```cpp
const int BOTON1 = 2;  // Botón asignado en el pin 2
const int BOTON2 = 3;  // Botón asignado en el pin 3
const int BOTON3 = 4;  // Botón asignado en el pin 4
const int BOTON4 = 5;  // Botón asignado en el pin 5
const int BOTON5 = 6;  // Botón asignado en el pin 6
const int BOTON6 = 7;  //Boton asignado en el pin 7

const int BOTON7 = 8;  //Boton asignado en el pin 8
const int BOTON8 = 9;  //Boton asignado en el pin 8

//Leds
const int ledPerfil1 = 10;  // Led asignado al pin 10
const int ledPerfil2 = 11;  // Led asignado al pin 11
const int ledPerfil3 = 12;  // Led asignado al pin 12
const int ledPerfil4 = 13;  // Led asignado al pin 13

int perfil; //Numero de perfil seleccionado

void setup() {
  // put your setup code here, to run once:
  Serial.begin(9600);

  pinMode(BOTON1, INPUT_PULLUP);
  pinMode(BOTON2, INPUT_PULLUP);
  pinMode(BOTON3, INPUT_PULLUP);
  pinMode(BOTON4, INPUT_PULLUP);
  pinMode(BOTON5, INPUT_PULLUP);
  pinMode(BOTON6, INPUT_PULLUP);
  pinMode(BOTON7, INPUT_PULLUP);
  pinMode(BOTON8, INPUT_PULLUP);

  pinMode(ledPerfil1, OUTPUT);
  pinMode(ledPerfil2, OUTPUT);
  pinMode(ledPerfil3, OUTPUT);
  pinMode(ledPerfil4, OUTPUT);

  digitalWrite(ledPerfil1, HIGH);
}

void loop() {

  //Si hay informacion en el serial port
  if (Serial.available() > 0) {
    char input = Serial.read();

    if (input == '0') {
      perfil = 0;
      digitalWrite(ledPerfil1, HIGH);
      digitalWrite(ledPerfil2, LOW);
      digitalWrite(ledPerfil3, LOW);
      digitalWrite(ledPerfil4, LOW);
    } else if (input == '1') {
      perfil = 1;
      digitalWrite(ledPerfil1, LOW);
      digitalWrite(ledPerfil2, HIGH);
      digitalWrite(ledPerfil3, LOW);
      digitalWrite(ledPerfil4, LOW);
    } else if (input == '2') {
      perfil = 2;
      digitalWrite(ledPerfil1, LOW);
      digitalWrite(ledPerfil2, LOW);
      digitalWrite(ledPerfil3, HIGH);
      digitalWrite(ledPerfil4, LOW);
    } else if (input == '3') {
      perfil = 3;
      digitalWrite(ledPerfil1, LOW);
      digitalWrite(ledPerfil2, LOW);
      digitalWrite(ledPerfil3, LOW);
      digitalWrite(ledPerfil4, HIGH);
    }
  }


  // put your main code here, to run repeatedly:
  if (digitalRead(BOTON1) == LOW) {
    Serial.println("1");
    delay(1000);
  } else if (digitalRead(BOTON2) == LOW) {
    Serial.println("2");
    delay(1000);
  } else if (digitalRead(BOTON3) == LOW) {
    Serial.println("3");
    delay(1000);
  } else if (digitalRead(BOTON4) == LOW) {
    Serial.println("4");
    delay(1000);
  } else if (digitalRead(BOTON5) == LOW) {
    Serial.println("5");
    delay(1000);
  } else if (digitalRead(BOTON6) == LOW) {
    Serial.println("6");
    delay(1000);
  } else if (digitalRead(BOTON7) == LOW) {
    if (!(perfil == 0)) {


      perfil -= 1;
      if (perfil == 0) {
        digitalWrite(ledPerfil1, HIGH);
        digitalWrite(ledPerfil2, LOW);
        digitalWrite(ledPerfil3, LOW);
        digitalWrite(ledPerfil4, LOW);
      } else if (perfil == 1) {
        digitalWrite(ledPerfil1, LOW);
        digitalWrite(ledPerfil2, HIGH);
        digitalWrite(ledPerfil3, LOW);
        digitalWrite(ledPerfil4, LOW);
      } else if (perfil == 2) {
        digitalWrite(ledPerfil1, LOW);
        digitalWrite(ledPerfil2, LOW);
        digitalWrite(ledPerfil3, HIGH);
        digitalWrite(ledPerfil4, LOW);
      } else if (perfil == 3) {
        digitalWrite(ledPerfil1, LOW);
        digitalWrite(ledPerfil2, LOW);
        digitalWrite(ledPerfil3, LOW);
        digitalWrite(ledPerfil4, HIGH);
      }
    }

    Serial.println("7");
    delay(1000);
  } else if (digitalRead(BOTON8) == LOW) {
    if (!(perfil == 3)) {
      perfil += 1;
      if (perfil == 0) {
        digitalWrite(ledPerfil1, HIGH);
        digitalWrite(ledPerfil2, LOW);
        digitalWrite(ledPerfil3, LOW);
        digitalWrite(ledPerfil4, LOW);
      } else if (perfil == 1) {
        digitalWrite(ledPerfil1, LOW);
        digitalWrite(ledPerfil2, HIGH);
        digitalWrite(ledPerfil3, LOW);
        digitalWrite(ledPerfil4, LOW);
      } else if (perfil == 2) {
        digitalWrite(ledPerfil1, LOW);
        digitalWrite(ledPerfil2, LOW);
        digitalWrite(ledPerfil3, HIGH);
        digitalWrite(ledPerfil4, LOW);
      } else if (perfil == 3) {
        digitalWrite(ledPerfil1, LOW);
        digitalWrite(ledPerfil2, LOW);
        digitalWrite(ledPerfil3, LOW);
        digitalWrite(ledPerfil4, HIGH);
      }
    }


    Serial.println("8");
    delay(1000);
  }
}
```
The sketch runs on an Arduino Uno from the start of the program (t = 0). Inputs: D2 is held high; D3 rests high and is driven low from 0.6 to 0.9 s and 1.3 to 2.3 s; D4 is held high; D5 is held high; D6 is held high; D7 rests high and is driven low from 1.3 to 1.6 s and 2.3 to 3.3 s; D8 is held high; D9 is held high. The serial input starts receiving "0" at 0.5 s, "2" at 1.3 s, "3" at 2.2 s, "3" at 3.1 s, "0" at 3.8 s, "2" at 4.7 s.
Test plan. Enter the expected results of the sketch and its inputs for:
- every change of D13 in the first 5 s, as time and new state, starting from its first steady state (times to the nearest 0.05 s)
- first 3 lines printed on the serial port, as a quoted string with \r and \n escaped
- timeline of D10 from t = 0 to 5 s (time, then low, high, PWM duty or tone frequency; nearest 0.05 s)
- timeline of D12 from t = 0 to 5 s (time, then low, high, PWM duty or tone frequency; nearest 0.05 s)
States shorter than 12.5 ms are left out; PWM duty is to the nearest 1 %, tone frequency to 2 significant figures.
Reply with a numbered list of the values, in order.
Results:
1. 0 s low; 2.6 s high; 3.8 s low
2. "2\r\n2\r\n6\r\n"
3. 0 s high; 1.6 s low; 3.8 s high; 4.7 s low
4. 0 s low; 1.6 s high; 2.6 s low; 4.7 s high
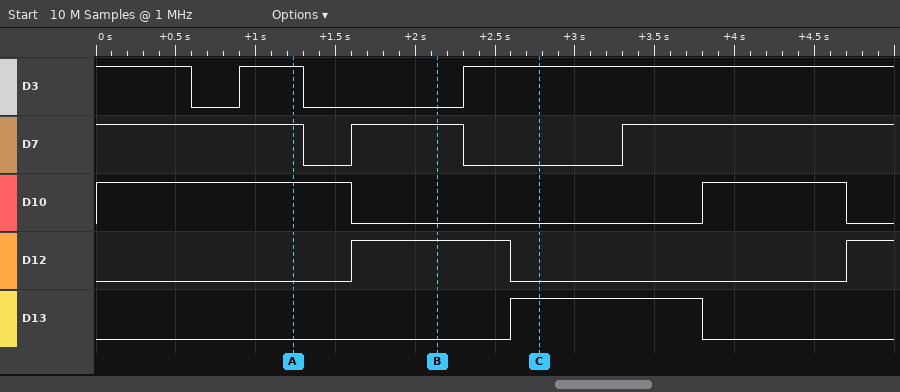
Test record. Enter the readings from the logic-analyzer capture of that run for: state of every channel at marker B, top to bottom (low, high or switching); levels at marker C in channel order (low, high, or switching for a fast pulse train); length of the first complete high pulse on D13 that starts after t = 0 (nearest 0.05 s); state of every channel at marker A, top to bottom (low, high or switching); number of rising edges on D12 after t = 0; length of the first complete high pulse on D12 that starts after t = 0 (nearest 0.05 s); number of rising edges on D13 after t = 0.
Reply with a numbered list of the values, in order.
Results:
1. D3 low, D7 high, D10 low, D12 high, D13 low
2. D3 high, D7 low, D10 low, D12 low, D13 high
3. 1.20 s
4. D3 high, D7 high, D10 high, D12 low, D13 low
5. 2
6. 1.00 s
7. 1
